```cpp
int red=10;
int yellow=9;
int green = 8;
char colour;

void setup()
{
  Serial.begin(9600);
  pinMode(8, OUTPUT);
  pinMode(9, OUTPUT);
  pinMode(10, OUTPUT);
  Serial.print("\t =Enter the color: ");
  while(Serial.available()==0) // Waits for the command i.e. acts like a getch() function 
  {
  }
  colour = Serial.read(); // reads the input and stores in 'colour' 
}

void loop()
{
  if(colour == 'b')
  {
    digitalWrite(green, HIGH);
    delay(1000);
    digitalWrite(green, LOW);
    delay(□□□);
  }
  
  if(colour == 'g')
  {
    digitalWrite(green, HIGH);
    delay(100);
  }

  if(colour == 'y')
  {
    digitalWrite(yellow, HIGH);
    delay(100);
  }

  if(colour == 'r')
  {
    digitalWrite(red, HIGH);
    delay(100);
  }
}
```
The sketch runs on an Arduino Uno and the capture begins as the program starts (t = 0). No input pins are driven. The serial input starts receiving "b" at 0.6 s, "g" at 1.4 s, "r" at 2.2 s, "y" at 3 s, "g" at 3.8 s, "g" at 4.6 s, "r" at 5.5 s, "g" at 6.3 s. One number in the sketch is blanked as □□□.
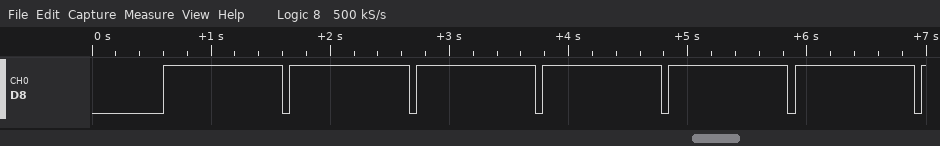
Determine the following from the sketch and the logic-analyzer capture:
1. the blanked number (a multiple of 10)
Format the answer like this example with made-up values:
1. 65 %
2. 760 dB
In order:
1. 60
